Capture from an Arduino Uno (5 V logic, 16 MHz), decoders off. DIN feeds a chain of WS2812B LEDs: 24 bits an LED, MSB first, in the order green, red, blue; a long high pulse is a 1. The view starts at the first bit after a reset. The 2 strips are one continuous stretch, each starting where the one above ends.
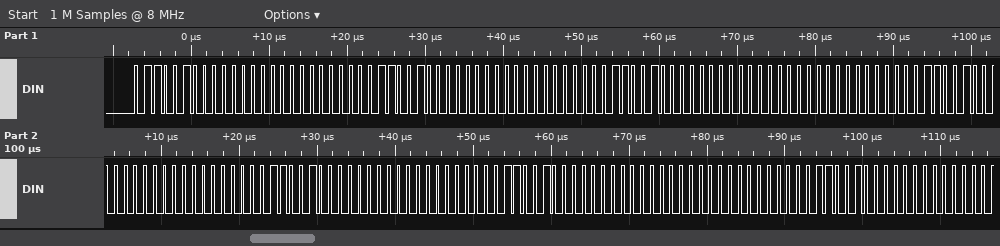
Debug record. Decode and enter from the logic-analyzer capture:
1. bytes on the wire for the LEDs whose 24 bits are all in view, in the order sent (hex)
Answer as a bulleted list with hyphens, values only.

- 64 00 00 64 00 00 64 00 00 00 64 00 00 64 00 00 64 00 00 00 64
